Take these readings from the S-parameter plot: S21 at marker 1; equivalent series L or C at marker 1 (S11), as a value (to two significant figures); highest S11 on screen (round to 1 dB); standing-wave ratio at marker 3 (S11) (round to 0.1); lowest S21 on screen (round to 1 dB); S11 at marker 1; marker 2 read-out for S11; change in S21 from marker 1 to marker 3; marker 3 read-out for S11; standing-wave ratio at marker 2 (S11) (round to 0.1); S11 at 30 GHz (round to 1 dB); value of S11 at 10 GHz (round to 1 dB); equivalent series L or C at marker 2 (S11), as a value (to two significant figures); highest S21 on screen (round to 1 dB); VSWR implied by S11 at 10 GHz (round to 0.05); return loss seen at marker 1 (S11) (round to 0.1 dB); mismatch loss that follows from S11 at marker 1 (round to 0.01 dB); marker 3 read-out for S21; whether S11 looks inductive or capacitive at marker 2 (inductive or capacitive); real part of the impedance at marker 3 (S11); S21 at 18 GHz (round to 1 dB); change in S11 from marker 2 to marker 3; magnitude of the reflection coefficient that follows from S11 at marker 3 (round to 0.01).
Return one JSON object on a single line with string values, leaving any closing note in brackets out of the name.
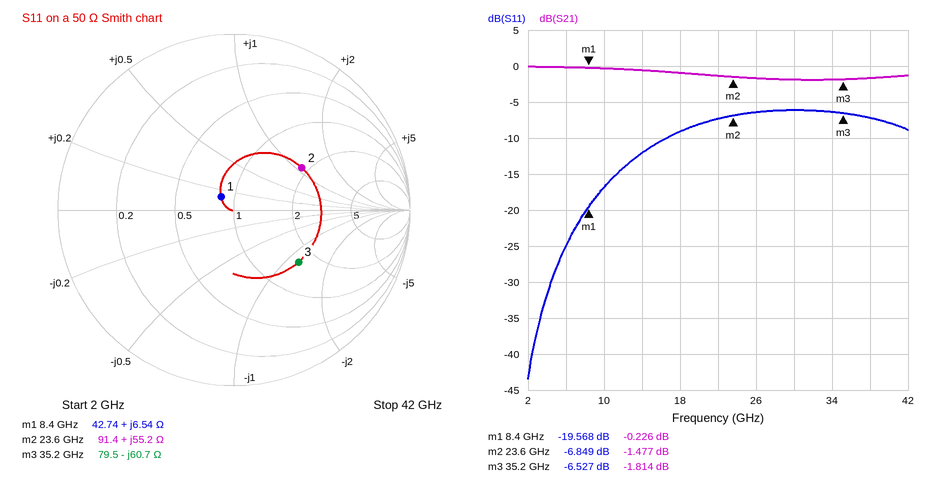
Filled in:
{"S21 at marker 1": "-0.226 dB", "equivalent series L or C at marker 1 (S11), as a value": "120 pH", "highest S11 on screen": "-6 dB", "standing-wave ratio at marker 3 (S11)": "2.8", "lowest S21 on screen": "-2 dB", "S11 at marker 1": "-19.568 dB", "marker 2 read-out for S11": "-6.849 dB", "change in S21 from marker 1 to marker 3": "-1.588 dB", "marker 3 read-out for S11": "-6.527 dB", "standing-wave ratio at marker 2 (S11)": "2.7", "S11 at 30 GHz": "-6 dB", "value of S11 at 10 GHz": "-17 dB", "equivalent series L or C at marker 2 (S11), as a value": "370 pH", "highest S21 on screen": "0 dB", "VSWR implied by S11 at 10 GHz": "1.35", "return loss seen at marker 1 (S11)": "19.6 dB", "mismatch loss that follows from S11 at marker 1": "0.05 dB", "marker 3 read-out for S21": "-1.814 dB", "whether S11 looks inductive or capacitive at marker 2": "inductive", "real part of the impedance at marker 3": "79.5 Ω", "S21 at 18 GHz": "-1 dB", "change in S11 from marker 2 to marker 3": "0.322 dB", "magnitude of the reflection coefficient that follows from S11 at marker 3": "0.47"}
